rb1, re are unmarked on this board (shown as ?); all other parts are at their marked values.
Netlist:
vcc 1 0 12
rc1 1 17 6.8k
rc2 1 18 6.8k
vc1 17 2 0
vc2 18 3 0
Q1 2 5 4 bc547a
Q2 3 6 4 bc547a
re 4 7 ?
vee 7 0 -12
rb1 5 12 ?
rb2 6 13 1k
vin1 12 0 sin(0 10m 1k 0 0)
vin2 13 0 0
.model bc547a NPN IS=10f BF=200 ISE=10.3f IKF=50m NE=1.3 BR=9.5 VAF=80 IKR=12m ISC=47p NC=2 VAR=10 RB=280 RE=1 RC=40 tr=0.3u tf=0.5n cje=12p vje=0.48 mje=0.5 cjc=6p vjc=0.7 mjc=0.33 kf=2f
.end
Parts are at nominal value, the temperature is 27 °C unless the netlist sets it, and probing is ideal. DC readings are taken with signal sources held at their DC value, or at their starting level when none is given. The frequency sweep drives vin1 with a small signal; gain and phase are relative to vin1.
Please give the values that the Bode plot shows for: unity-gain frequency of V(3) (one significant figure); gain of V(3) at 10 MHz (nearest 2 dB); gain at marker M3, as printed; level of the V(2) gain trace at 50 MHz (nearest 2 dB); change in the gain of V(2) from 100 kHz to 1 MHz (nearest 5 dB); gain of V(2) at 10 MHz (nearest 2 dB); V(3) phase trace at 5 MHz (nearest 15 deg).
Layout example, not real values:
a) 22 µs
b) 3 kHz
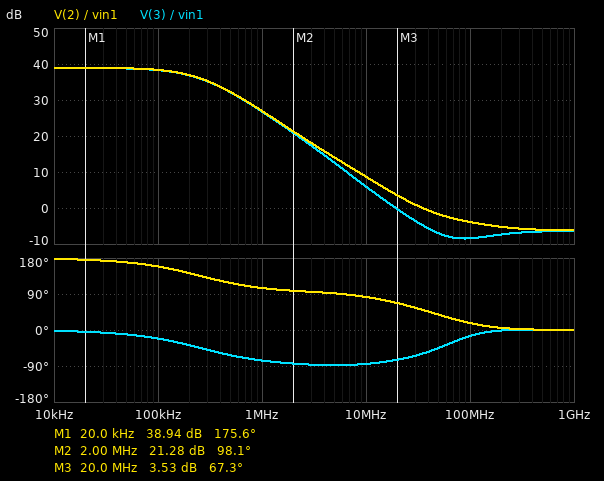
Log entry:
a) 20 MHz
b) 6 dB
c) 3.53 dB
d) -2 dB
e) -10 dB
f) 8 dB
g) -90 deg
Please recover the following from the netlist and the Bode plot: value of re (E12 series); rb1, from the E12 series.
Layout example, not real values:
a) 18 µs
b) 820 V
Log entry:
a) 5.6 kΩ
b) 560 Ω
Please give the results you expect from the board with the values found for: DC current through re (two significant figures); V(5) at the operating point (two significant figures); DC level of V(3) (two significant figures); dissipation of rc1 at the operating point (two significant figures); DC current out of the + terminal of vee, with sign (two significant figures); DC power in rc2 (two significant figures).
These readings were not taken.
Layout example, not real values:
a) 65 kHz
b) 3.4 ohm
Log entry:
a) 2.0 mA
b) -4.8 mV
c) 5.5 V
d) 7.5 mW
e) -2.0 mA
f) 6.2 mW
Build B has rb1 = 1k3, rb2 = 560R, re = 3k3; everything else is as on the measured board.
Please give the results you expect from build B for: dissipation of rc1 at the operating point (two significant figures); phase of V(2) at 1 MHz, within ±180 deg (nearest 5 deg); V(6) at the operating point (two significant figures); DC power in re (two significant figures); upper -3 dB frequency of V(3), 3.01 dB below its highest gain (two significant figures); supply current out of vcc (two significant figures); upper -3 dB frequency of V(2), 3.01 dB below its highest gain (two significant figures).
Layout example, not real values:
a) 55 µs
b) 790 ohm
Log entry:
a) 17 mW
b) 140 deg
c) -10 mV
d) 39 mW
e) 110 kHz
f) 3.4 mA
g) 140 kHz
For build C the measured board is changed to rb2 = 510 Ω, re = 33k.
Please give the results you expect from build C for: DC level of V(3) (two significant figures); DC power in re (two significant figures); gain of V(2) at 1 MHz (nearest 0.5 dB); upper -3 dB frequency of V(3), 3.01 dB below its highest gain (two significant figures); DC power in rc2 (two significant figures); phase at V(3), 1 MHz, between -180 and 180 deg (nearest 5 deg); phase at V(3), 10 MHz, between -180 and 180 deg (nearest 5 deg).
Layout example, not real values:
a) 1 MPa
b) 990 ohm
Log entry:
a) 11 V
b) 3.9 mW
c) 24.5 dB
d) 1.3 MHz
e) 200 µW
f) -40 deg
g) -90 deg
